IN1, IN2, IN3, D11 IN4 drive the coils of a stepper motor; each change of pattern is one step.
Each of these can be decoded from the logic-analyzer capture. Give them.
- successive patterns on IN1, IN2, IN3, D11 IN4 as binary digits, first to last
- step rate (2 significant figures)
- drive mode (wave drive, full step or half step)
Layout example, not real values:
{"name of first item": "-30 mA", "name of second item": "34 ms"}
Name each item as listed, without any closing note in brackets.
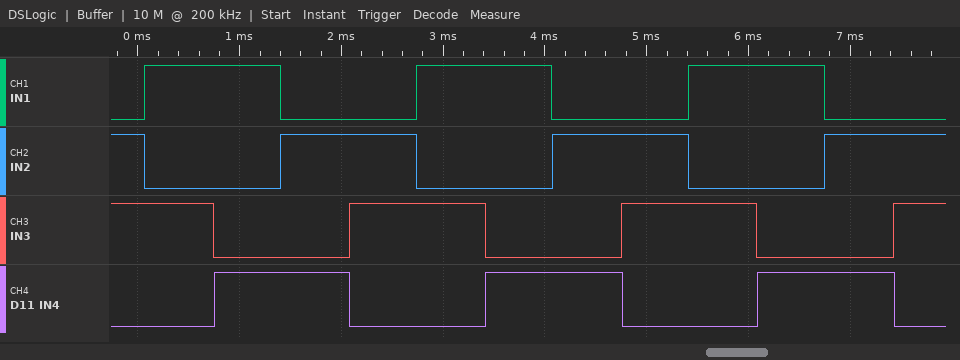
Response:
{"successive patterns on IN1, IN2, IN3, D11 IN4 as binary digits, first to last": "0110 1010 1001 0101 0110 1010 1001 0101 0110 1010 1001 0101 0110", "step rate": "1500 steps/s", "drive mode": "full step"}
